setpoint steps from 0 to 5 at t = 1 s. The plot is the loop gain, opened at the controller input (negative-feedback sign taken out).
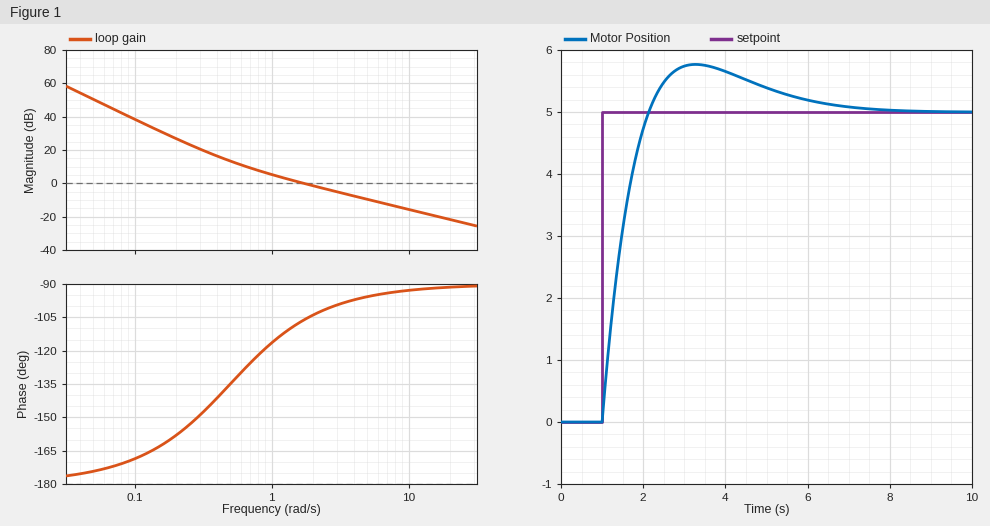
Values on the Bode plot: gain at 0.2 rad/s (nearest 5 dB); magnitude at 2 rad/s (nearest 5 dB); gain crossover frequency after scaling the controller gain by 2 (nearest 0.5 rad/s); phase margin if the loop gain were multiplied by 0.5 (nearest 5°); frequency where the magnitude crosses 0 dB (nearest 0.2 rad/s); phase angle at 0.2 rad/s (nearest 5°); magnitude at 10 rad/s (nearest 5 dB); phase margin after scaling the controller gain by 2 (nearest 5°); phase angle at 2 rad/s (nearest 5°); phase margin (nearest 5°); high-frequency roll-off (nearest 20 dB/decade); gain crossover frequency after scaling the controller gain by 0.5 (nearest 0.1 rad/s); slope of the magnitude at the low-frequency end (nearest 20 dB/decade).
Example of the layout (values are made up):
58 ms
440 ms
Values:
25 dB
0 dB
3.5 rad/s
60°
1.8 rad/s
-160°
-15 dB
80°
-105°
75°
-20 dB/decade
0.9 rad/s
-40 dB/decade
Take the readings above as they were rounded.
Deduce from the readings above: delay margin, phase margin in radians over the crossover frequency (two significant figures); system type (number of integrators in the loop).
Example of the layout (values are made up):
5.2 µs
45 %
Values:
0.73 s
2
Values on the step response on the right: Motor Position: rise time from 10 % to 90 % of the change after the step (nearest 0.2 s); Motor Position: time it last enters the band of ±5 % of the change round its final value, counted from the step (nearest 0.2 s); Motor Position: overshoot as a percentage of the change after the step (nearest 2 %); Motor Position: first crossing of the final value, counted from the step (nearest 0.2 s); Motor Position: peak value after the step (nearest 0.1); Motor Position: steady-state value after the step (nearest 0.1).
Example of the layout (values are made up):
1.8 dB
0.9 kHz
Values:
0.8 s
4.6 s
16 %
1.2 s
5.8
5.0
